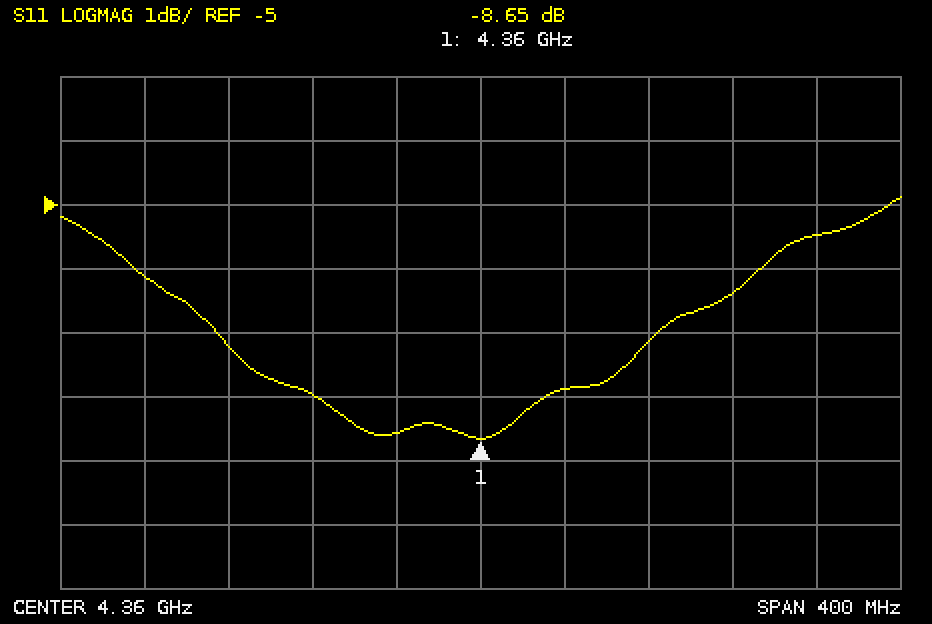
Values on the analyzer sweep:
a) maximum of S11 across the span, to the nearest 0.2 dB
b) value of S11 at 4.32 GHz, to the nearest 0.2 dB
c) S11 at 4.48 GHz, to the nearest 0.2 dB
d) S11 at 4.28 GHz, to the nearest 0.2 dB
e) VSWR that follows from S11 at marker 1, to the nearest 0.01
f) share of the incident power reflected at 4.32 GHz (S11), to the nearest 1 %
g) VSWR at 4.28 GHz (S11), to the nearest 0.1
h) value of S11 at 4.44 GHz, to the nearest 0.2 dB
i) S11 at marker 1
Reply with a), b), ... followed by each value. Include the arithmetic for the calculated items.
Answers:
a) -4.8 dB
b) -8.6 dB
c) -6.4 dB
d) -8.0 dB
e) (1 + 0.3694)/(1 − 0.3694) ≈ 2.17
f) 10^(-8.6/10) ≈ 14 %
g) |Γ| = 10^(-8/20) = 0.3981; VSWR = (1 + 0.3981)/(1 − 0.3981) ≈ 2.3
h) -7.2 dB
i) -8.65 dB
